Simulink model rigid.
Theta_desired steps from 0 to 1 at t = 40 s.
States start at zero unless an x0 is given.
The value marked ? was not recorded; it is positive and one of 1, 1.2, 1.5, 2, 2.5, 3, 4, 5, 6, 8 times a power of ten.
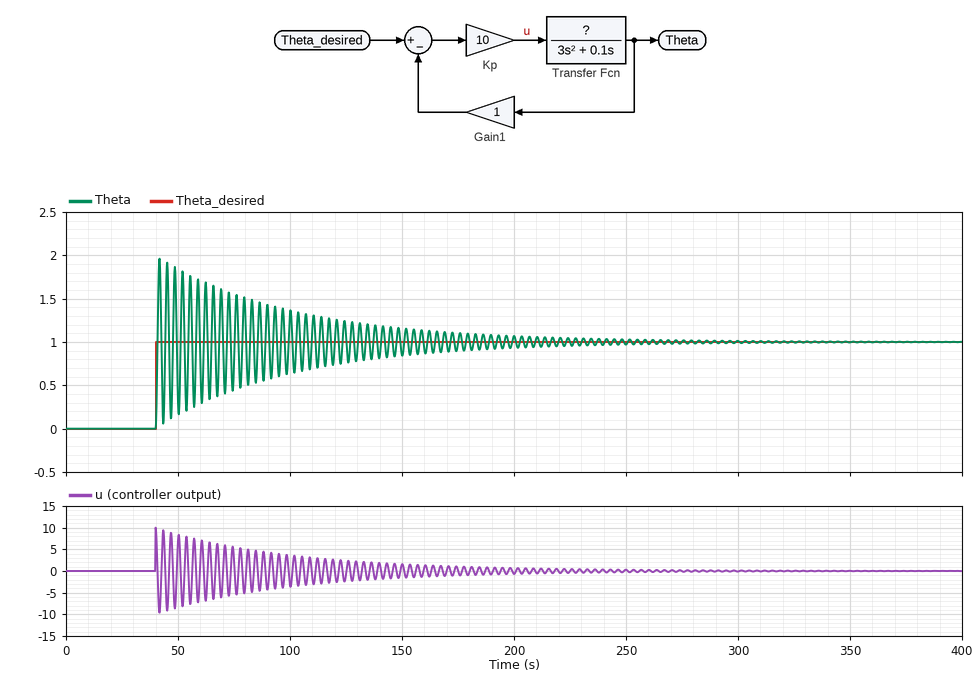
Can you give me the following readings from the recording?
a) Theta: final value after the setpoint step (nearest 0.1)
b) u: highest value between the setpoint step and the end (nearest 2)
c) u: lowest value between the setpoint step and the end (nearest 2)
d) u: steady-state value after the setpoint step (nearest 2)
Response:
1.0
10
-10
0
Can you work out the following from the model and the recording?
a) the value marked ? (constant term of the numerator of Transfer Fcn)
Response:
1
